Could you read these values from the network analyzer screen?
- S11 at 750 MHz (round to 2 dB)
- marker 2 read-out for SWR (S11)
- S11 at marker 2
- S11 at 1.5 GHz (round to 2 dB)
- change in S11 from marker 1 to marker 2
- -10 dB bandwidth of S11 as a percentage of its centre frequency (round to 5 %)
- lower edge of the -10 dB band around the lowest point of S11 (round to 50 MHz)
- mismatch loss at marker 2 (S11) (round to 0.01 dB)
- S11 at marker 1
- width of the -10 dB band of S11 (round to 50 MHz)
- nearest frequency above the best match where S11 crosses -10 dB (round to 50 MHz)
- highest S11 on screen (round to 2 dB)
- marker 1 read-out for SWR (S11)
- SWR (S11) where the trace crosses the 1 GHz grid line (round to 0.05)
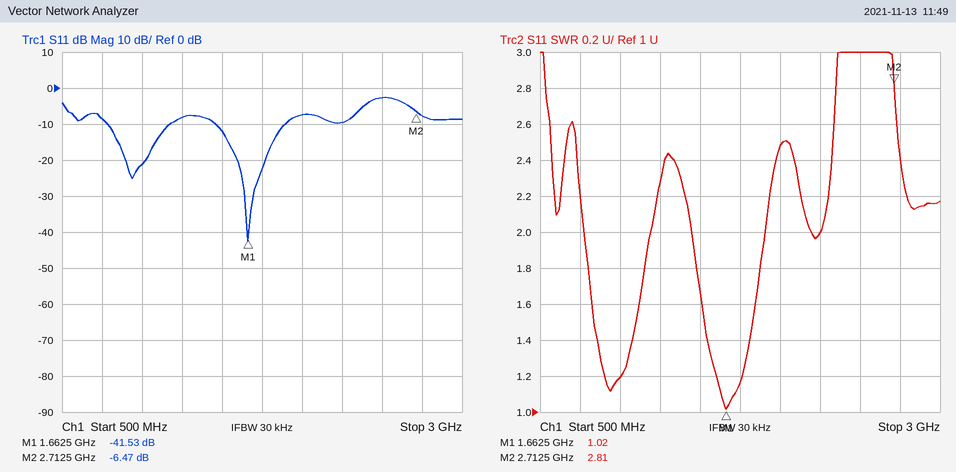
-8 dB
2.81
-6.47 dB
-12 dB
35.06 dB
25 %
1.45 GHz
1.11 dB
-41.53 dB
450 MHz
1.90 GHz
-2 dB
1.02
1.20
